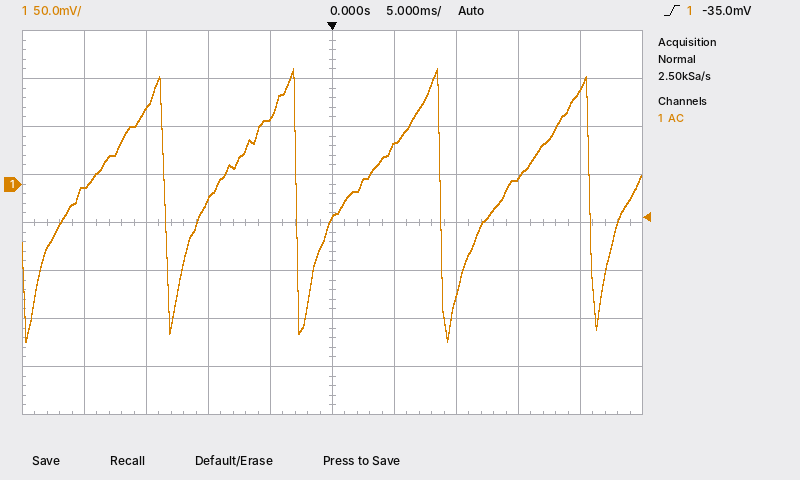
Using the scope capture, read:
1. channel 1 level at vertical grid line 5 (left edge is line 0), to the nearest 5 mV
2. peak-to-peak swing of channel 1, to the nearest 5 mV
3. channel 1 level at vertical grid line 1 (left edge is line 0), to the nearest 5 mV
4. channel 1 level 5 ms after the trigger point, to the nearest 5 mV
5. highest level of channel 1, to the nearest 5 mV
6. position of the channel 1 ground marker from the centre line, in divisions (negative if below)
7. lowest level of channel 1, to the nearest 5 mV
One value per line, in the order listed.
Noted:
-35 mV
285 mV
-5 mV
40 mV
120 mV
+0.8 div
-165 mV
